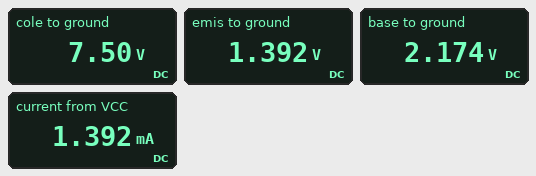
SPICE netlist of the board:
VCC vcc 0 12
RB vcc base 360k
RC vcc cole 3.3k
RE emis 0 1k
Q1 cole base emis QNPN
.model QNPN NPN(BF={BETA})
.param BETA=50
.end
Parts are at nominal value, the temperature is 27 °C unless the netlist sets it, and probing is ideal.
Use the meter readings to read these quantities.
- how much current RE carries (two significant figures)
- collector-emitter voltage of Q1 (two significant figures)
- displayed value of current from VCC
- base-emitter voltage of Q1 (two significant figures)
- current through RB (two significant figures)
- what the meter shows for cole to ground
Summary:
1.4 mA
6.1 V
1.392 mA
780 mV
27 µA
7.50 V
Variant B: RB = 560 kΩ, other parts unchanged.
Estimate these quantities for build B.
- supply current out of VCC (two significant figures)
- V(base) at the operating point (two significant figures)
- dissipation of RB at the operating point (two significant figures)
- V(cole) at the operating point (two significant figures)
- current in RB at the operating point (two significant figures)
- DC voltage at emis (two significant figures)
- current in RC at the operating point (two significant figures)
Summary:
940 µA
1.7 V
190 µW
9.0 V
18 µA
940 mV
920 µA
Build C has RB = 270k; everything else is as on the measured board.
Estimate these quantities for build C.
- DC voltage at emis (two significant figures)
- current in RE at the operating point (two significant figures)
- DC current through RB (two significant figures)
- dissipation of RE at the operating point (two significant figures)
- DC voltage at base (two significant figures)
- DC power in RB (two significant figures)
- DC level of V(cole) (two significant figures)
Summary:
1.8 V
1.8 mA
35 µA
3.2 mW
2.6 V
330 µW
6.2 V
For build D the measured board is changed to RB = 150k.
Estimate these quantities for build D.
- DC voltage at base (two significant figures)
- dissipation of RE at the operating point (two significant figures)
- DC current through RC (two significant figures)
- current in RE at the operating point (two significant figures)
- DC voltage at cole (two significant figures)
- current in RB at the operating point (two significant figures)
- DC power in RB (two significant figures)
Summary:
3.6 V
7.8 mW
2.7 mA
2.8 mA
3.0 V
56 µA
470 µW
